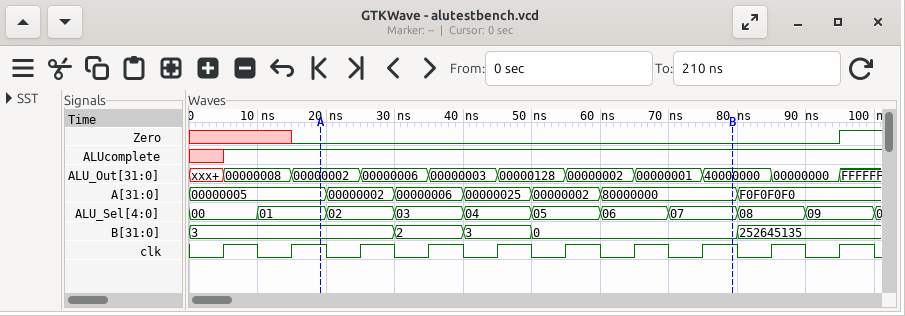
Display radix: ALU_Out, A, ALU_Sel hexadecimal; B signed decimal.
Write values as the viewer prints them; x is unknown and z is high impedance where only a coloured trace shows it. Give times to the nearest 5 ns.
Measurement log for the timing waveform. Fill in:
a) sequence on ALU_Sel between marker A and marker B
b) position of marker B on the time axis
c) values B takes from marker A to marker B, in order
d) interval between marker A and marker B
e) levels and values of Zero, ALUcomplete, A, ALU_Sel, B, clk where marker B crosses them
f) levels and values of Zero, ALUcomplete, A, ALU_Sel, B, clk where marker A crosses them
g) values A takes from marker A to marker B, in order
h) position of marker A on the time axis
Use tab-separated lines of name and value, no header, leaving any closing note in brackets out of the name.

sequence on ALU_Sel between marker A and marker B	01, 02, 03, 04, 05, 06, 07
position of marker B on the time axis	80 ns
values B takes from marker A to marker B, in order	3, 2, 3, 0
interval between marker A and marker B	60 ns
levels and values of Zero, ALUcomplete, A, ALU_Sel, B, clk where marker B crosses them	Zero=0, ALUcomplete=1, A=80000000, ALU_Sel=07, B=0, clk=1
levels and values of Zero, ALUcomplete, A, ALU_Sel, B, clk where marker A crosses them	Zero=0, ALUcomplete=1, A=00000005, ALU_Sel=01, B=3, clk=1
values A takes from marker A to marker B, in order	00000005, 00000002, 00000006, 00000025, 00000002, 80000000
position of marker A on the time axis	20 ns
